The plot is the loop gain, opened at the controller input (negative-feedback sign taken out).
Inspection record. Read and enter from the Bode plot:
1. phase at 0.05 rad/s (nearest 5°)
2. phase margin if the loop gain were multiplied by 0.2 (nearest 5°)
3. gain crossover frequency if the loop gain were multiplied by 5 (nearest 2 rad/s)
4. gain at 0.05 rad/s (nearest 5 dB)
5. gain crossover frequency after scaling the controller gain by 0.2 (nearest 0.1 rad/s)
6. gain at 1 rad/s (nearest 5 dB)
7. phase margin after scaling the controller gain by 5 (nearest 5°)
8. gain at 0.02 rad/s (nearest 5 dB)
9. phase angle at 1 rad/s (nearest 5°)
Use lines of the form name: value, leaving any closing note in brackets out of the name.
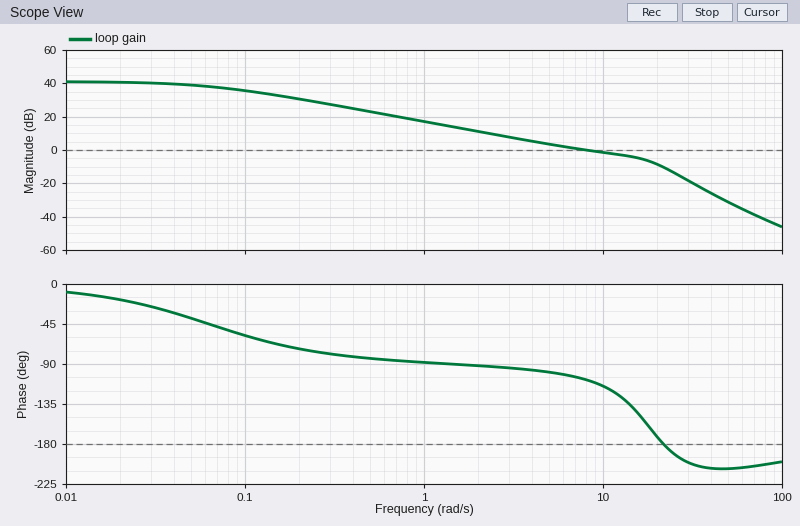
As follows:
phase at 0.05 rad/s: -40°
phase margin if the loop gain were multiplied by 0.2: 90°
gain crossover frequency if the loop gain were multiplied by 5: 26 rad/s
gain at 0.05 rad/s: 40 dB
gain crossover frequency after scaling the controller gain by 0.2: 1.4 rad/s
gain at 1 rad/s: 15 dB
phase margin after scaling the controller gain by 5: -10°
gain at 0.02 rad/s: 40 dB
phase angle at 1 rad/s: -90°
